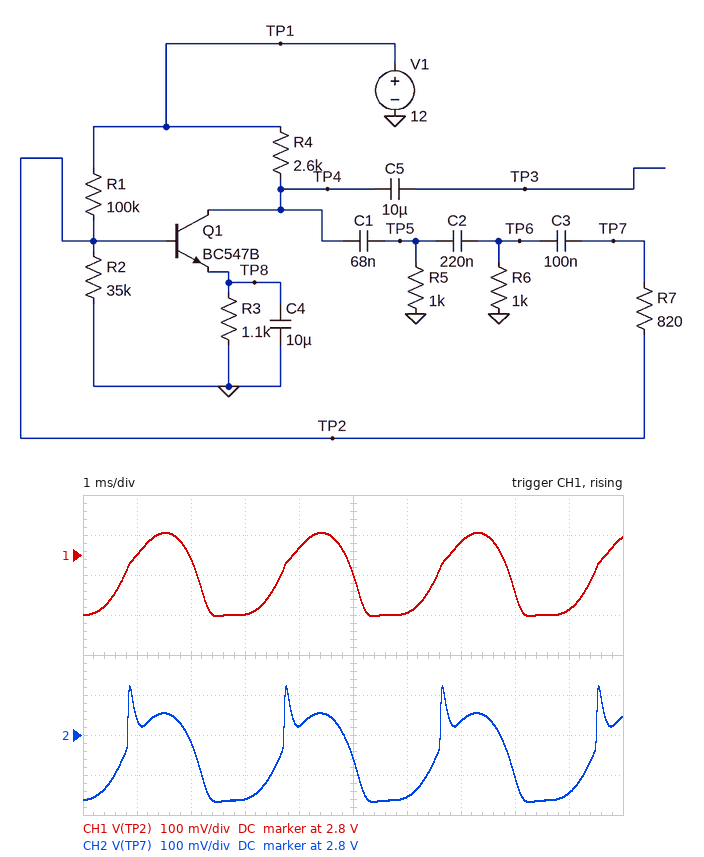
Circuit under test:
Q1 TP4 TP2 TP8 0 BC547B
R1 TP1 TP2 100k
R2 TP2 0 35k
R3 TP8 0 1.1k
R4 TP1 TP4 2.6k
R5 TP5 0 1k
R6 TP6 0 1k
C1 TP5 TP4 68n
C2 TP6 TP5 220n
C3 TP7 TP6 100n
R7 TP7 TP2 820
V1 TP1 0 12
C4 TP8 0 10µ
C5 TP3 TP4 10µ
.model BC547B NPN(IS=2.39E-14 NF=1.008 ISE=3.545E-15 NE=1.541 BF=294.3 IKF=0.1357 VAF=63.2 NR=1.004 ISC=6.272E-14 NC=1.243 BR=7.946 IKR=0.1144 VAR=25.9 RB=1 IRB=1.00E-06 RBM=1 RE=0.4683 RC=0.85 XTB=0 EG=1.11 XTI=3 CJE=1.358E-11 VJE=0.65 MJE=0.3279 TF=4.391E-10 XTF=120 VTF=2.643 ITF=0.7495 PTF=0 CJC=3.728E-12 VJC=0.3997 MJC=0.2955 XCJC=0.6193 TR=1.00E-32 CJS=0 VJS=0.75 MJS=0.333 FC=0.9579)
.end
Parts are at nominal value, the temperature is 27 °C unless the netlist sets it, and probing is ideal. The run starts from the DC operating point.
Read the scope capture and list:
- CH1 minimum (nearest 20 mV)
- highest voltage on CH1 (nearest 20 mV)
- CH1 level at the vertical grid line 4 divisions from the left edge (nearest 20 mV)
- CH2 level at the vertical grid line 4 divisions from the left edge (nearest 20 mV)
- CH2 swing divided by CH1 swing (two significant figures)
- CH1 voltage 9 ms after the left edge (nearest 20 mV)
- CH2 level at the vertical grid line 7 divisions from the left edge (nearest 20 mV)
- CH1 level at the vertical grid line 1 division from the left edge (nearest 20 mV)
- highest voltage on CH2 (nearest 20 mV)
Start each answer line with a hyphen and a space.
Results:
- 2.64 V
- 2.86 V
- 2.82 V
- 2.82 V
- 1.4
- 2.66 V
- 2.84 V
- 2.80 V
- 2.92 V
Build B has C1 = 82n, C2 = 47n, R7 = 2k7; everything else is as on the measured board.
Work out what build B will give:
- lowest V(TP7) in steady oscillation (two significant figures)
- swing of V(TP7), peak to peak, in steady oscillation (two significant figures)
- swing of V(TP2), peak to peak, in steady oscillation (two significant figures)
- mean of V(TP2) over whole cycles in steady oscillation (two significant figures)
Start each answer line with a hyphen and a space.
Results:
- 2.8 V
- 240 mV
- 160 mV
- 2.9 V
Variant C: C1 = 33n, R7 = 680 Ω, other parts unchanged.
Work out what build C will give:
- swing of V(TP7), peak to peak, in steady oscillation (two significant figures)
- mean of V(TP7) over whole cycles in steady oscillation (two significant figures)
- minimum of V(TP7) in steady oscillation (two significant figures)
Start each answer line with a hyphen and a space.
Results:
- 190 mV
- 2.8 V
- 2.7 V
